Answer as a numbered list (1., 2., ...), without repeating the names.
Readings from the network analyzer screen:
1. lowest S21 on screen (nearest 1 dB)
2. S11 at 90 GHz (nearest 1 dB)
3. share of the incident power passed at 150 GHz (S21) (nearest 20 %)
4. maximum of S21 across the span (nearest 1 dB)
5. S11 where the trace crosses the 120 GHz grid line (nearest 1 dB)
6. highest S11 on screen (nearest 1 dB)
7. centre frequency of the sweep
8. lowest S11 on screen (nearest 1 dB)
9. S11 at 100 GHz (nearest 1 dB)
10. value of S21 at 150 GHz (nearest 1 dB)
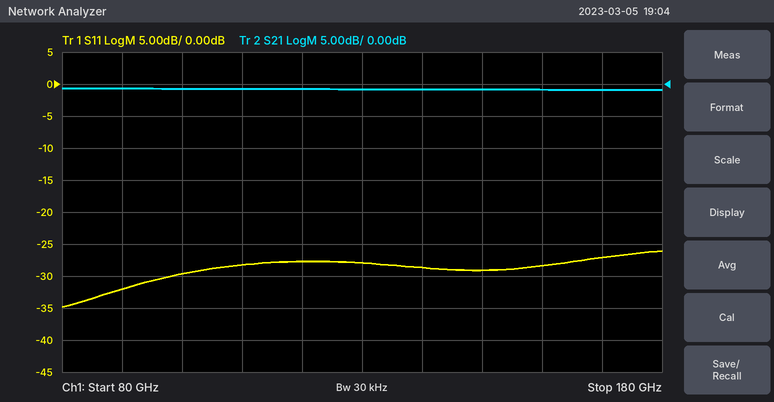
1. -1 dB
2. -32 dB
3. 80 %
4. -1 dB
5. -28 dB
6. -26 dB
7. 130 GHz
8. -35 dB
9. -30 dB
10. -1 dB
